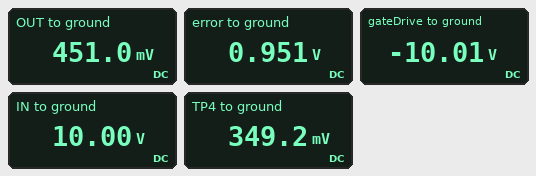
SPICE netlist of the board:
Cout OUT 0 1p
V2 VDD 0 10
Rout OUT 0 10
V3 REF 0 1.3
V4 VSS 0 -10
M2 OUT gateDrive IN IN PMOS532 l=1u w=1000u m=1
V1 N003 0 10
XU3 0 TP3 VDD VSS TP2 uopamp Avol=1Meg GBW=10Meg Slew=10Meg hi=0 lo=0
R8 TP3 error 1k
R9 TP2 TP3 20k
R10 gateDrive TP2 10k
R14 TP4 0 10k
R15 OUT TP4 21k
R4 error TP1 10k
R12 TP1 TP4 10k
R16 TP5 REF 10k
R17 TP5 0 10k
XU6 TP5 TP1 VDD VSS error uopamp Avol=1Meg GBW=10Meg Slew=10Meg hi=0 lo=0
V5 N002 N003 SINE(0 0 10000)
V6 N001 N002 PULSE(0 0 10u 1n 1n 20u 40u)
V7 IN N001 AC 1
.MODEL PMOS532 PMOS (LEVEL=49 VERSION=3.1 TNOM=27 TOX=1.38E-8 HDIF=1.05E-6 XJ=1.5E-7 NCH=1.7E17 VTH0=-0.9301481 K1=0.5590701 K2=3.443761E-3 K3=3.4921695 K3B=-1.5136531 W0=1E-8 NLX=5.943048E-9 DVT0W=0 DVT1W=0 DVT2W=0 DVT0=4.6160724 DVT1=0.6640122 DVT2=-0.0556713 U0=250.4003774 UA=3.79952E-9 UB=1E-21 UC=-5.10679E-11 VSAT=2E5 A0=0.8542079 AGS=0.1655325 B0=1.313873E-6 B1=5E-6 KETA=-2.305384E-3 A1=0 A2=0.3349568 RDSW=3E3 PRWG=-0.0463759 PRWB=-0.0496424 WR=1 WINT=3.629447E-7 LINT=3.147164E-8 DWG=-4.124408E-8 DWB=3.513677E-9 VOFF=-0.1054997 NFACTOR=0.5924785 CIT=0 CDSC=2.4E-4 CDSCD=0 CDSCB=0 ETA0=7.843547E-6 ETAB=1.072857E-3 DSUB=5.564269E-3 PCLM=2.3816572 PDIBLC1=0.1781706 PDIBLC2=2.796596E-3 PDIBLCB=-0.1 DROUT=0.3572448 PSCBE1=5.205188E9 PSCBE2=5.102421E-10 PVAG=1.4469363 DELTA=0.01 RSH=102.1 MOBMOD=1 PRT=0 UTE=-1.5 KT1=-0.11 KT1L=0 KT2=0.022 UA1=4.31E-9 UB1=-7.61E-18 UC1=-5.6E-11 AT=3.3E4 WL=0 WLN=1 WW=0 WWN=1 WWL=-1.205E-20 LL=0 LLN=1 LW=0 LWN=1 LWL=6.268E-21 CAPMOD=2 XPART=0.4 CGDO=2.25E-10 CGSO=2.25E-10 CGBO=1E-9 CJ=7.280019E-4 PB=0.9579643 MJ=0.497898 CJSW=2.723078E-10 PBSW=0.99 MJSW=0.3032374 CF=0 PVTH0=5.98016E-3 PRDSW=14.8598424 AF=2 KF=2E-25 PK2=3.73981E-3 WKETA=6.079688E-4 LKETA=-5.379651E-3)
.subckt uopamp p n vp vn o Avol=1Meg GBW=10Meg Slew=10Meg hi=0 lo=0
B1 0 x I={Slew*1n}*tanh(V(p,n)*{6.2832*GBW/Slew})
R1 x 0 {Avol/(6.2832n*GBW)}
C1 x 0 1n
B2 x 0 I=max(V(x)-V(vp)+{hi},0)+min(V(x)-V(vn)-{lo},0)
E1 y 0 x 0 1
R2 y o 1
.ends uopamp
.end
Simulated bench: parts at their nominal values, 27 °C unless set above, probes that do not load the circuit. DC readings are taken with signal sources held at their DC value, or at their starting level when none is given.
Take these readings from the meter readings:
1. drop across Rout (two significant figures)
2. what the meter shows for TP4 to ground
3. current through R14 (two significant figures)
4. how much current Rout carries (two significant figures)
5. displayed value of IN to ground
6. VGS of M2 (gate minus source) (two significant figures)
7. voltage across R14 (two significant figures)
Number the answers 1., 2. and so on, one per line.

1. 450 mV
2. 349.2 mV
3. 35 µA
4. 45 mA
5. 10.00 V
6. -20 V
7. 350 mV
